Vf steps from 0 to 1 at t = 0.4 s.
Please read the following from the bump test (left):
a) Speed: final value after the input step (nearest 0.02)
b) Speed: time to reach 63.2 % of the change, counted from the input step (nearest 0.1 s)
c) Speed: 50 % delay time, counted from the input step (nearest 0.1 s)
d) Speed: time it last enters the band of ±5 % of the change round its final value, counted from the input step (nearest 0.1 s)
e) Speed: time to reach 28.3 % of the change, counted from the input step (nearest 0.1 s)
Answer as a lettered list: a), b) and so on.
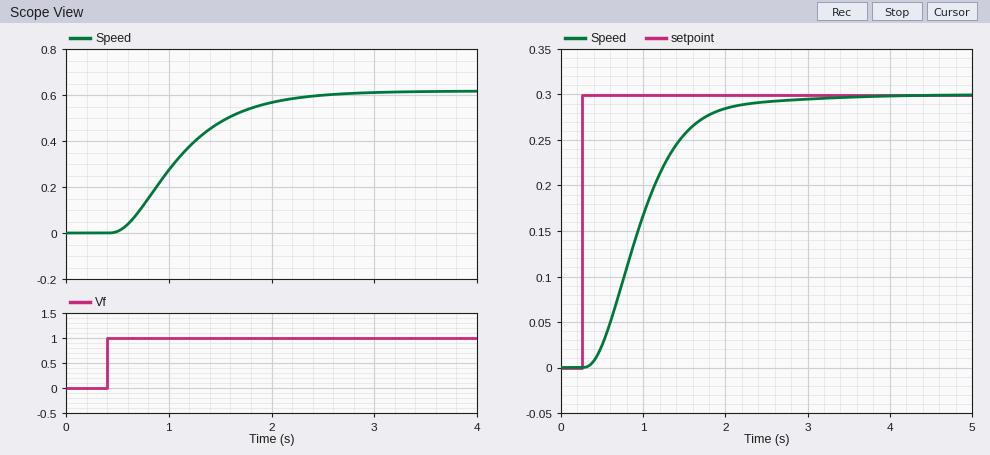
a) 0.62
b) 0.8 s
c) 0.7 s
d) 1.8 s
e) 0.4 s
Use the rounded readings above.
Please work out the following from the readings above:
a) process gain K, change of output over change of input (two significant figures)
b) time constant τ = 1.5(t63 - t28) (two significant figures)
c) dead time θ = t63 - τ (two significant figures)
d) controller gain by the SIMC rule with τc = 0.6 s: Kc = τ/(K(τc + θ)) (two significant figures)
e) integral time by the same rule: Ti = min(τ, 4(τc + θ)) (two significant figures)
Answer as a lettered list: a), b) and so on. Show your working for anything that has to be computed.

a) (0.62 - 0) / 1 = 0.62
b) 1.5 × (0.8 - 0.4) = 0.60 s
c) 0.8 - 0.6 = 0.20 s
d) 0.6 / (0.62 × (0.6 + 0.2)) = 1.2
e) min(0.6, 4 × (0.6 + 0.2)) = 0.60 s
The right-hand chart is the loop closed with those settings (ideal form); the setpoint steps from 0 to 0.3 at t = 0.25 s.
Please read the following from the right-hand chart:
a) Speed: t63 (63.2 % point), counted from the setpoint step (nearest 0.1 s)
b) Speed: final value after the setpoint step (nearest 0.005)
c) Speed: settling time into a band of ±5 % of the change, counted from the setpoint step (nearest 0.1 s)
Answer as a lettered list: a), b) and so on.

a) 0.8 s
b) 0.300
c) 1.8 s
